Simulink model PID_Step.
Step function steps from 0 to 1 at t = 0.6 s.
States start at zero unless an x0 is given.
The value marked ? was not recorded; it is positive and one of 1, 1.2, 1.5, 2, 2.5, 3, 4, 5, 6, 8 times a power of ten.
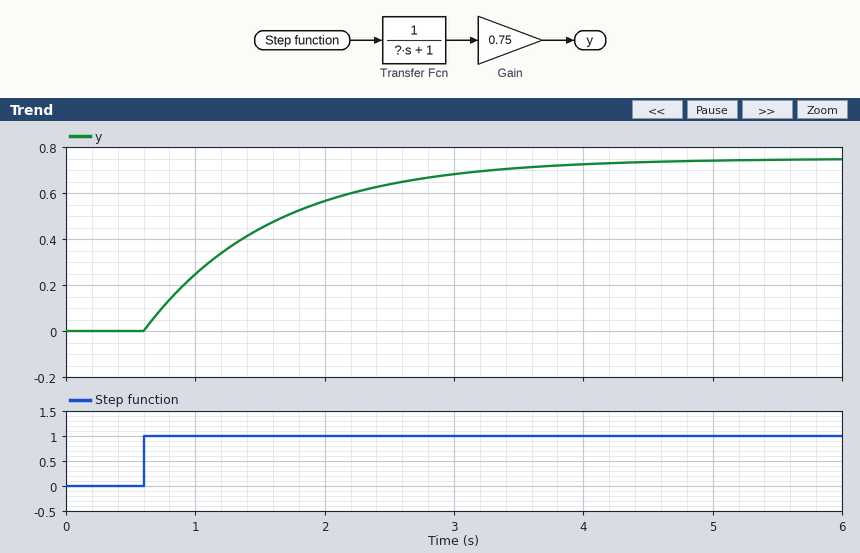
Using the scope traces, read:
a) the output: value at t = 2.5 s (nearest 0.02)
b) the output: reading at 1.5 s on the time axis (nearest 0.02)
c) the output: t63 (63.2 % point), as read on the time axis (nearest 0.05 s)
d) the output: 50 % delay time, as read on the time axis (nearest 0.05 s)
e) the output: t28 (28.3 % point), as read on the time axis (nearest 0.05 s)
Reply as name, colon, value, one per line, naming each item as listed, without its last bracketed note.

the output: value at t = 2.5 s: 0.64
the output: reading at 1.5 s on the time axis: 0.44
the output: t63 (63.2 % point), as read on the time axis: 1.60 s
the output: 50 % delay time, as read on the time axis: 1.30 s
the output: t28 (28.3 % point), as read on the time axis: 0.95 s
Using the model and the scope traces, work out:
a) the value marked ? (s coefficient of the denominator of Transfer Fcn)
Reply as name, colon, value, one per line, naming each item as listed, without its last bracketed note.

the value marked ?: 1
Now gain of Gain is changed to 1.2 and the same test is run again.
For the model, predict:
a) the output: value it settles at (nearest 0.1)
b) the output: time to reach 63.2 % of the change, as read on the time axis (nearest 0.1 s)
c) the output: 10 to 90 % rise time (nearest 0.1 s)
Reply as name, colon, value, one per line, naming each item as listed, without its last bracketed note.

the output: value it settles at: 1.2
the output: time to reach 63.2 % of the change, as read on the time axis: 1.6 s
the output: 10 to 90 % rise time: 2.2 s
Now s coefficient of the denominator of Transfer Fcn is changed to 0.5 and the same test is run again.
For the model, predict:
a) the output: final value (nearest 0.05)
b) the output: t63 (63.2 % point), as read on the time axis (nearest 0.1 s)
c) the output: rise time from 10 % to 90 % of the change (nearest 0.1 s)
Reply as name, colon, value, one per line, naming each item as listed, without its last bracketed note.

the output: final value: 0.75
the output: t63 (63.2 % point), as read on the time axis: 1.1 s
the output: rise time from 10 % to 90 % of the change: 1.1 s
